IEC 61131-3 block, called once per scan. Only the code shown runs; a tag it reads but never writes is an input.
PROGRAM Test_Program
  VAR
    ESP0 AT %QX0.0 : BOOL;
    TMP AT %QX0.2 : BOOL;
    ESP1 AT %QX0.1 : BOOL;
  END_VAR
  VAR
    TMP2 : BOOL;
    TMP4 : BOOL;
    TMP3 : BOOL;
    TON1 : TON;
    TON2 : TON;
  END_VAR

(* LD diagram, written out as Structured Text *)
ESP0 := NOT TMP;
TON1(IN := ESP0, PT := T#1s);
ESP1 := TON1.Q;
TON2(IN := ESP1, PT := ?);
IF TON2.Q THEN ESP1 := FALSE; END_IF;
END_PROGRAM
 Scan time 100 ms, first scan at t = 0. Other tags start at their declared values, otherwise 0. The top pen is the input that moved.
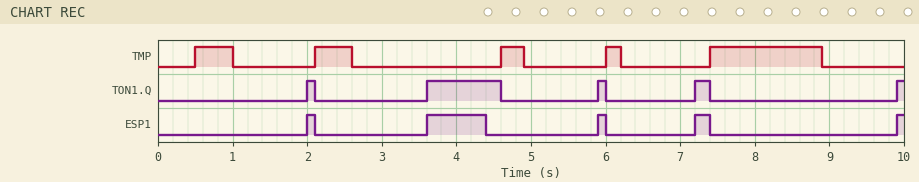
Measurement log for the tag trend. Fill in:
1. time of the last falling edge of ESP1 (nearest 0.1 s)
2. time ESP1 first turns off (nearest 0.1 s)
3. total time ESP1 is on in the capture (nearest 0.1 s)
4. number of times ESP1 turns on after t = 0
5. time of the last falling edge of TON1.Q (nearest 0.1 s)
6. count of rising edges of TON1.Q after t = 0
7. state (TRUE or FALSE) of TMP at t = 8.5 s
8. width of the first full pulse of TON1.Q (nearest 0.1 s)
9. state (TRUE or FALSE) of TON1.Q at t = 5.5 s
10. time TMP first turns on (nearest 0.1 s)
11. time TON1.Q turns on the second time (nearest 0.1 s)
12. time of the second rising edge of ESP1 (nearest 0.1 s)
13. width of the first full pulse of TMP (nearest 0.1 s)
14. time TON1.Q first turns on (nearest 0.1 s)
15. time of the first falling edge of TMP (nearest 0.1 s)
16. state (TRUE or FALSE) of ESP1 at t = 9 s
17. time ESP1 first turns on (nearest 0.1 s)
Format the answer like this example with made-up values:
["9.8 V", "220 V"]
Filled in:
["7.4 s", "2.1 s", "1.3 s", "5", "7.4 s", "5", "TRUE", "0.1 s", "FALSE", "0.5 s", "3.6 s", "3.6 s", "0.5 s", "2.0 s", "1.0 s", "FALSE", "2.0 s"]
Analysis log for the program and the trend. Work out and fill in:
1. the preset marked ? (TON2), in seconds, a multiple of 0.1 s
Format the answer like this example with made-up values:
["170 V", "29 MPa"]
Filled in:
["0.8 s"]
